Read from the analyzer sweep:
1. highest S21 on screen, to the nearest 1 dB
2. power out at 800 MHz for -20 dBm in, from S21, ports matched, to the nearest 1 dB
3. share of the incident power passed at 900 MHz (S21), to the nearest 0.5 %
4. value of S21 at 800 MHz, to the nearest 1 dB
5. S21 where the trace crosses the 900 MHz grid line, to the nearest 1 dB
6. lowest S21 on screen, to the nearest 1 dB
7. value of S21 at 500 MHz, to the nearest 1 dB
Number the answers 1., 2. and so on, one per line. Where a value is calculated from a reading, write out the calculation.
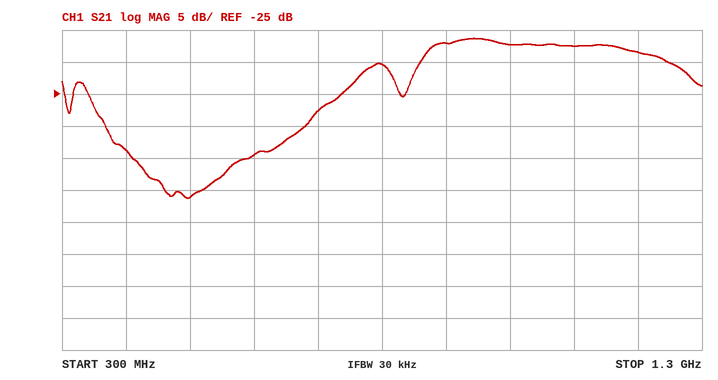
1. -16 dB
2. -20 dBm + (-20 dB) = -40 dBm
3. 10^(-17/10) ≈ 2.0 %
4. -20 dB
5. -17 dB
6. -41 dB
7. -41 dB
